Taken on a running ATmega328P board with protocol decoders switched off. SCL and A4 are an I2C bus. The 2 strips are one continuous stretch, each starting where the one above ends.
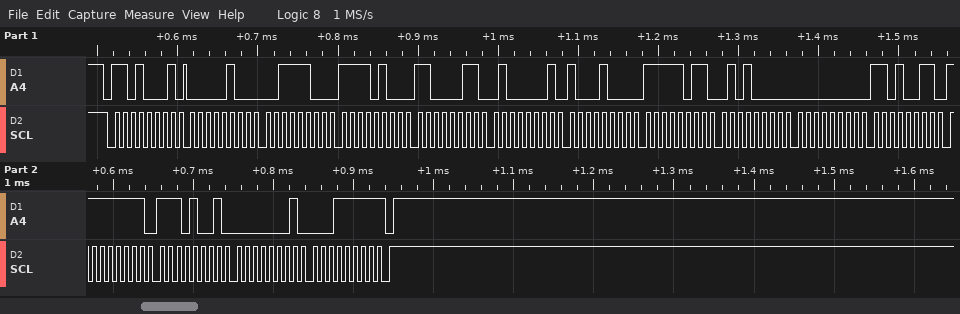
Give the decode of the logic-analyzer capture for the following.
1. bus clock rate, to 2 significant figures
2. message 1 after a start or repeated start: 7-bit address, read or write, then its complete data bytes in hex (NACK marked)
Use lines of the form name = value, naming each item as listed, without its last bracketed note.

bus clock rate, to 2 significant figures = 100 kHz
message 1 after a start or repeated start: 7-bit address, read or write, then its complete data bytes in hex = 0x68 read: 04 3C F4 C3 41 88 FB 50 00 D3 FF E9 01 1F NACK
